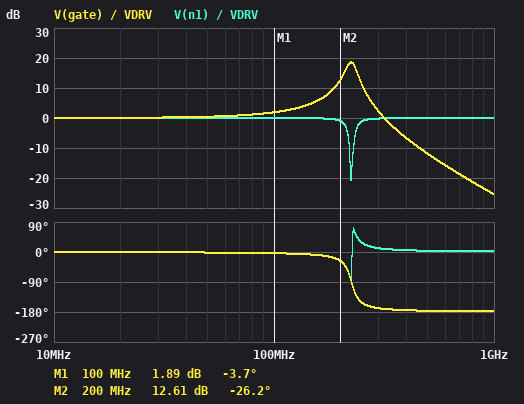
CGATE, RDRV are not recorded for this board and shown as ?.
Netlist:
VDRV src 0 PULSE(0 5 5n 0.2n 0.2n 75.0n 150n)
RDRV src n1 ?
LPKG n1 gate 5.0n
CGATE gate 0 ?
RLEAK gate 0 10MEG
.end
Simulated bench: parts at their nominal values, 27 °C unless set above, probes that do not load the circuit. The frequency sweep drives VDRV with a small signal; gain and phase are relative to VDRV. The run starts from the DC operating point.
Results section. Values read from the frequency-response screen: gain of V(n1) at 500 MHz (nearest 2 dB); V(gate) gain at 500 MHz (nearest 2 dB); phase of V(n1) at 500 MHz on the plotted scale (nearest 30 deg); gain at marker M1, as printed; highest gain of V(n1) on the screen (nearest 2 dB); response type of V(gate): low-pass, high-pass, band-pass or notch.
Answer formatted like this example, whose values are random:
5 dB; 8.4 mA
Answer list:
0 dB; -12 dB; 0 deg; 1.89 dB; 0 dB; low-pass
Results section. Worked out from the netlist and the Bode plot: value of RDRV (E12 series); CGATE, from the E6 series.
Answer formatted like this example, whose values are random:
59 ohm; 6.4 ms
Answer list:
0.82 Ω; 100 pF
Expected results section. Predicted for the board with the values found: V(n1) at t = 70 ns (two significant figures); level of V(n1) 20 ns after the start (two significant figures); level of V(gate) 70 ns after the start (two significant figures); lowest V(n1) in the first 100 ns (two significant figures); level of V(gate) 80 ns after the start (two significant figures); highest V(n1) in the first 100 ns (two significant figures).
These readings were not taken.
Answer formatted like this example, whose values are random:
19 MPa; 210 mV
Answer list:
5.0 V; 4.9 V; 5.0 V; -440 mV; 5.0 V; 5.4 V
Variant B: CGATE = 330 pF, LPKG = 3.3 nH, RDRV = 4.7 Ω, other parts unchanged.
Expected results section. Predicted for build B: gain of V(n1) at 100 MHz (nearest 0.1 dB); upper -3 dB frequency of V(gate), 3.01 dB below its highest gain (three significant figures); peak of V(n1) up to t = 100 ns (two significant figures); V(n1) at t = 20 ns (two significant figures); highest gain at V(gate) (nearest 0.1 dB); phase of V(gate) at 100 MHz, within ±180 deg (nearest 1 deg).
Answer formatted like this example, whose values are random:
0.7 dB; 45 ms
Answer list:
-5.9 dB; 145 MHz; 5.1 V; 5.0 V; 0 dB; -60 deg
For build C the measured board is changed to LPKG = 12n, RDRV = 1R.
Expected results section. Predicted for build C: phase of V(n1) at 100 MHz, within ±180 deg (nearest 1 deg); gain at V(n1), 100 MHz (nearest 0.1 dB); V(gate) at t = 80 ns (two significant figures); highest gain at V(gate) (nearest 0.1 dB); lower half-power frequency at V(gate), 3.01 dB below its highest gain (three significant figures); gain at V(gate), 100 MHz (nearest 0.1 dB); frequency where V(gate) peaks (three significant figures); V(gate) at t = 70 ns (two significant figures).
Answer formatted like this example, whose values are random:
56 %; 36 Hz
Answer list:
-7 deg; -0.1 dB; 4.9 V; 20.8 dB; 138 MHz; 5.5 dB; 145 MHz; 5.3 V
